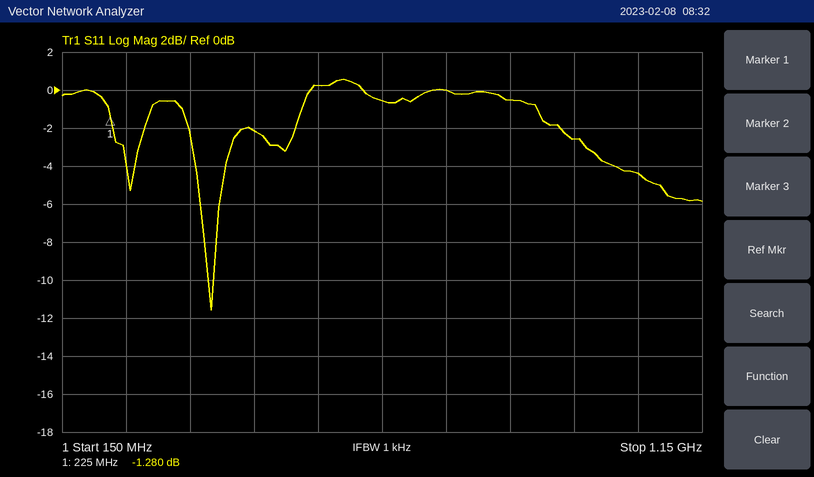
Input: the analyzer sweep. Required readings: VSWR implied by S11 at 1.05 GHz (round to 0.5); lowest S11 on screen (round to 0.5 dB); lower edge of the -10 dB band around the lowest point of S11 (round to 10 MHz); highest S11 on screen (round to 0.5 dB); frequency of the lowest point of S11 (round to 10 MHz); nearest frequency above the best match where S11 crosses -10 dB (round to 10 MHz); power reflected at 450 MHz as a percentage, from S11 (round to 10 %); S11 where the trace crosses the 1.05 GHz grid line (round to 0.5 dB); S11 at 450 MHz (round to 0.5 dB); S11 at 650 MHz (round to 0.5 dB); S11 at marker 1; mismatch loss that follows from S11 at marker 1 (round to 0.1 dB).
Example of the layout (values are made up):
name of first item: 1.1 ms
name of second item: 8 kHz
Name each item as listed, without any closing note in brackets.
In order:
VSWR implied by S11 at 1.05 GHz: 4.0
lowest S11 on screen: -11.5 dB
lower edge of the -10 dB band around the lowest point of S11: 380 MHz
highest S11 on screen: 0.5 dB
frequency of the lowest point of S11: 380 MHz
nearest frequency above the best match where S11 crosses -10 dB: 390 MHz
power reflected at 450 MHz as a percentage, from S11: 60 %
S11 where the trace crosses the 1.05 GHz grid line: -4.5 dB
S11 at 450 MHz: -2.0 dB
S11 at 650 MHz: -0.5 dB
S11 at marker 1: -1.280 dB
mismatch loss that follows from S11 at marker 1: 5.9 dB
